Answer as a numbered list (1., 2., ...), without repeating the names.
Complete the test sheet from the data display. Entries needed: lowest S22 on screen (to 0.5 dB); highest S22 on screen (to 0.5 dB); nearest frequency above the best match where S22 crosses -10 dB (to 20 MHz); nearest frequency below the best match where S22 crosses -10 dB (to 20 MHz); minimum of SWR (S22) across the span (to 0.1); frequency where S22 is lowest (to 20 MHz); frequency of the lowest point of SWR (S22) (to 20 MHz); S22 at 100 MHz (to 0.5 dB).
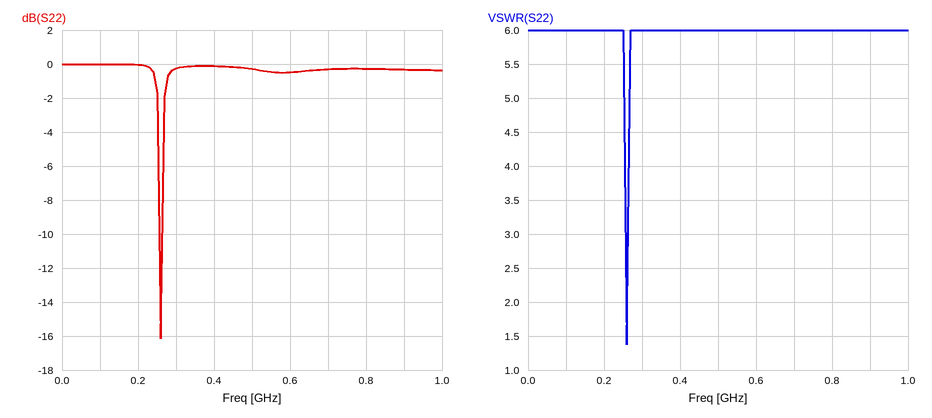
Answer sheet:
1. -16.0 dB
2. 0.0 dB
3. 260 MHz
4. 260 MHz
5. 1.4
6. 260 MHz
7. 260 MHz
8. 0.0 dB
